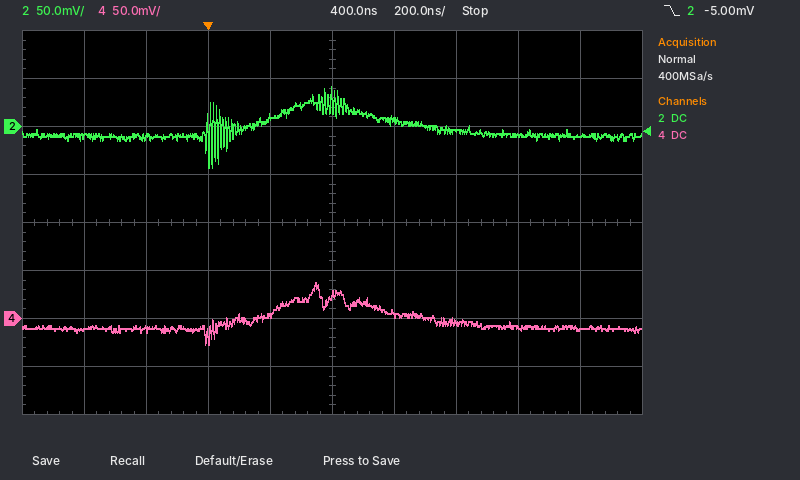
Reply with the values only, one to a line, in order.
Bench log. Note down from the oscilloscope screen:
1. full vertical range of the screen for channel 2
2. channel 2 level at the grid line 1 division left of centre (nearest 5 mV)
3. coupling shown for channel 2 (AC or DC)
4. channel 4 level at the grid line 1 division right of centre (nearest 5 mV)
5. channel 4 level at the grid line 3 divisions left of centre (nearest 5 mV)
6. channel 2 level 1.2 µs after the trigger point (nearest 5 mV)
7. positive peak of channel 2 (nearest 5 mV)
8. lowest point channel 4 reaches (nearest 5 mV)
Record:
400 mV
10 mV
DC
5 mV
-10 mV
-10 mV
40 mV
-25 mV
